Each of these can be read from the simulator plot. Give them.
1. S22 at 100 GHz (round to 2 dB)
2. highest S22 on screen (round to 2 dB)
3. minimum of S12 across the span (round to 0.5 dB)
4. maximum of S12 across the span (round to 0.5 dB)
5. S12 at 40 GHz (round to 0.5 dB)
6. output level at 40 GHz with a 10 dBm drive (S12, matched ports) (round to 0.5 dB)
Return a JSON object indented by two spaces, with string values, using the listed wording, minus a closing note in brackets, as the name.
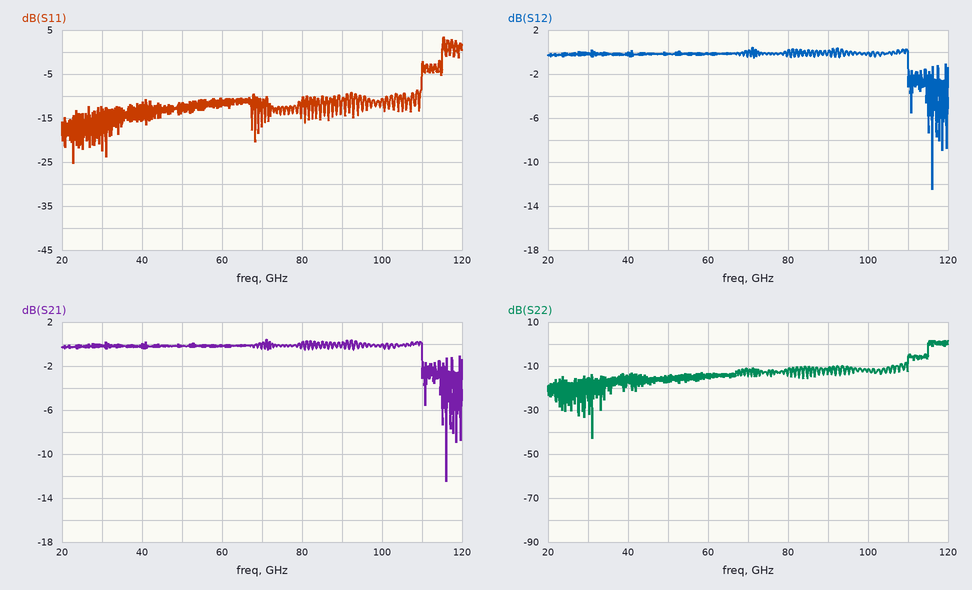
{
  "S22 at 100 GHz": "-12 dB",
  "highest S22 on screen": "2 dB",
  "minimum of S12 across the span": "-12.5 dB",
  "maximum of S12 across the span": "0.5 dB",
  "S12 at 40 GHz": "0.0 dB",
  "output level at 40 GHz with a 10 dBm drive (S12, matched ports)": "10.0 dBm"
}
